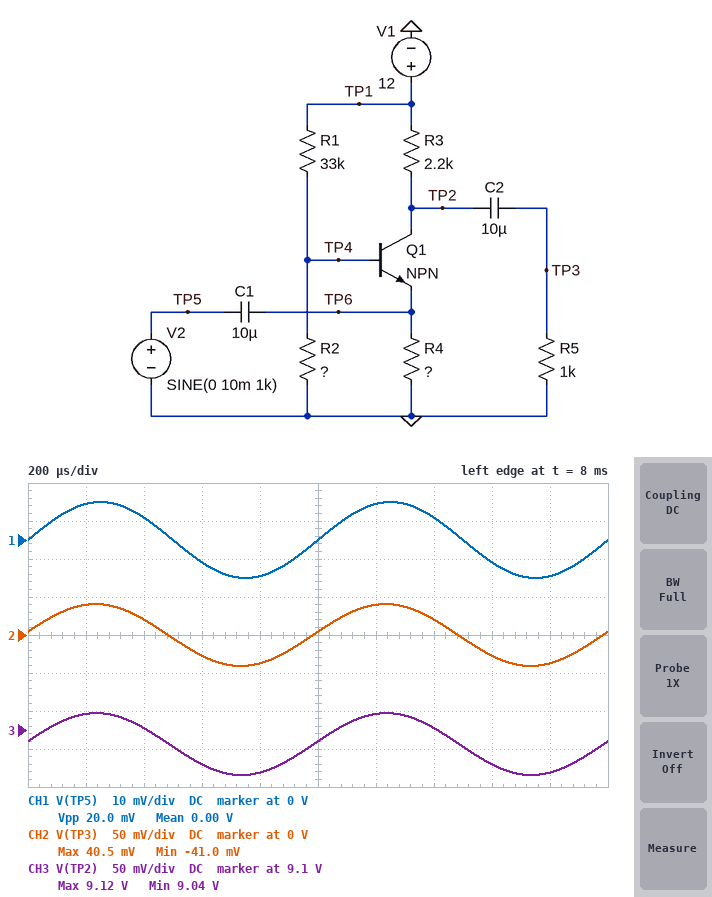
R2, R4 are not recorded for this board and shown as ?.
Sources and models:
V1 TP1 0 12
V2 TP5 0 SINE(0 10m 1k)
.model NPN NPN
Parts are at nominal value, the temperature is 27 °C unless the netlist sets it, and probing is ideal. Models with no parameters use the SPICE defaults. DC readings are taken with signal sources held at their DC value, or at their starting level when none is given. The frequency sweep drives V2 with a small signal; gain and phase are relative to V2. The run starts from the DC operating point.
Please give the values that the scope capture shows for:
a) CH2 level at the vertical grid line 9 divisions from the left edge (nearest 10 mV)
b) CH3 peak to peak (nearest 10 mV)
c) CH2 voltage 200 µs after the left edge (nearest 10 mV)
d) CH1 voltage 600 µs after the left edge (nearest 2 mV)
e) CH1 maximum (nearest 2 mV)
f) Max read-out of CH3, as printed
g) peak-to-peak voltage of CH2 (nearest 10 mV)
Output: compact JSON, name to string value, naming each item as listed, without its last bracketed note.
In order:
{"CH2 level at the vertical grid line 9 divisions from the left edge": "-40 mV", "CH3 peak to peak": "80 mV", "CH2 voltage 200 µs after the left edge": "40 mV", "CH1 voltage 600 µs after the left edge": "-6 mV", "CH1 maximum": "10 mV", "Max read-out of CH3, as printed": "9.12 V", "peak-to-peak voltage of CH2": "80 mV"}
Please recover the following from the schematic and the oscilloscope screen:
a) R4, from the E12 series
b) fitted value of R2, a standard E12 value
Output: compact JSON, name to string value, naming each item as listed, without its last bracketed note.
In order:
{"R4, from the E12 series": "3.3 kΩ", "fitted value of R2, a standard E12 value": "27 kΩ"}
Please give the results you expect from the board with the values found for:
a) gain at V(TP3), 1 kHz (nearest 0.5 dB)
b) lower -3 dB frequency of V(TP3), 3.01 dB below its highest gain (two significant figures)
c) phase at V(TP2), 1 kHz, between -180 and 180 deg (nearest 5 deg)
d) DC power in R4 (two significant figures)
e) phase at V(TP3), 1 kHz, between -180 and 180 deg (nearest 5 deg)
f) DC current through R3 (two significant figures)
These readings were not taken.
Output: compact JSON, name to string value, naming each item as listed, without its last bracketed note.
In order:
{"gain at V(TP3), 1 kHz": "12.0 dB", "lower -3 dB frequency of V(TP3), 3.01 dB below its highest gain": "100 Hz", "phase at V(TP2), 1 kHz, between -180 and 180 deg": "5 deg", "DC power in R4": "5.9 mW", "phase at V(TP3), 1 kHz, between -180 and 180 deg": "5 deg", "DC current through R3": "1.3 mA"}
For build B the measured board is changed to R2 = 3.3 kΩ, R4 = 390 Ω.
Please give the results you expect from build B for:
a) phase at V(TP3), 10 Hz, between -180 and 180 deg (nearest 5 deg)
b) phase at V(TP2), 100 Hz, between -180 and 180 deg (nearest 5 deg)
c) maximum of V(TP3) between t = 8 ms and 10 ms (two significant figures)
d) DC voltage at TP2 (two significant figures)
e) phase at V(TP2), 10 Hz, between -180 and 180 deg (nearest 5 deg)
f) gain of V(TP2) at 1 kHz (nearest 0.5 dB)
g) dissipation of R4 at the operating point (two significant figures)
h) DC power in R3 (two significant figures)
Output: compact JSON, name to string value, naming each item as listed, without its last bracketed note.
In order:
{"phase at V(TP3), 10 Hz, between -180 and 180 deg": "115 deg", "phase at V(TP2), 100 Hz, between -180 and 180 deg": "65 deg", "maximum of V(TP3) between t = 8 ms and 10 ms": "100 mV", "DC voltage at TP2": "10 V", "phase at V(TP2), 10 Hz, between -180 and 180 deg": "55 deg", "gain of V(TP2) at 1 kHz": "20.5 dB", "dissipation of R4 at the operating point": "230 µW", "DC power in R3": "1.3 mW"}
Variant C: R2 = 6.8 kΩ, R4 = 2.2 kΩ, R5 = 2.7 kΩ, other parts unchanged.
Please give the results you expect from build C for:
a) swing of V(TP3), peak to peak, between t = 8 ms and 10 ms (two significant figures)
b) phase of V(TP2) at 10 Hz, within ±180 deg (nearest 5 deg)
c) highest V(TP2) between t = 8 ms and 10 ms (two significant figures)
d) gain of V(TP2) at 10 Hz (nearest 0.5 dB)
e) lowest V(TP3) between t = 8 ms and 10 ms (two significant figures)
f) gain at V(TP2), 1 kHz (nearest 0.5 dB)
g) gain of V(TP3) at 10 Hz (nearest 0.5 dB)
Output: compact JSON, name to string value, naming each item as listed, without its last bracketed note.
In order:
{"swing of V(TP3), peak to peak, between t = 8 ms and 10 ms": "230 mV", "phase of V(TP2) at 10 Hz, within ±180 deg": "75 deg", "highest V(TP2) between t = 8 ms and 10 ms": "11 V", "gain of V(TP2) at 10 Hz": "-2.0 dB", "lowest V(TP3) between t = 8 ms and 10 ms": "-120 mV", "gain at V(TP2), 1 kHz": "21.5 dB", "gain of V(TP3) at 10 Hz": "-3.5 dB"}
